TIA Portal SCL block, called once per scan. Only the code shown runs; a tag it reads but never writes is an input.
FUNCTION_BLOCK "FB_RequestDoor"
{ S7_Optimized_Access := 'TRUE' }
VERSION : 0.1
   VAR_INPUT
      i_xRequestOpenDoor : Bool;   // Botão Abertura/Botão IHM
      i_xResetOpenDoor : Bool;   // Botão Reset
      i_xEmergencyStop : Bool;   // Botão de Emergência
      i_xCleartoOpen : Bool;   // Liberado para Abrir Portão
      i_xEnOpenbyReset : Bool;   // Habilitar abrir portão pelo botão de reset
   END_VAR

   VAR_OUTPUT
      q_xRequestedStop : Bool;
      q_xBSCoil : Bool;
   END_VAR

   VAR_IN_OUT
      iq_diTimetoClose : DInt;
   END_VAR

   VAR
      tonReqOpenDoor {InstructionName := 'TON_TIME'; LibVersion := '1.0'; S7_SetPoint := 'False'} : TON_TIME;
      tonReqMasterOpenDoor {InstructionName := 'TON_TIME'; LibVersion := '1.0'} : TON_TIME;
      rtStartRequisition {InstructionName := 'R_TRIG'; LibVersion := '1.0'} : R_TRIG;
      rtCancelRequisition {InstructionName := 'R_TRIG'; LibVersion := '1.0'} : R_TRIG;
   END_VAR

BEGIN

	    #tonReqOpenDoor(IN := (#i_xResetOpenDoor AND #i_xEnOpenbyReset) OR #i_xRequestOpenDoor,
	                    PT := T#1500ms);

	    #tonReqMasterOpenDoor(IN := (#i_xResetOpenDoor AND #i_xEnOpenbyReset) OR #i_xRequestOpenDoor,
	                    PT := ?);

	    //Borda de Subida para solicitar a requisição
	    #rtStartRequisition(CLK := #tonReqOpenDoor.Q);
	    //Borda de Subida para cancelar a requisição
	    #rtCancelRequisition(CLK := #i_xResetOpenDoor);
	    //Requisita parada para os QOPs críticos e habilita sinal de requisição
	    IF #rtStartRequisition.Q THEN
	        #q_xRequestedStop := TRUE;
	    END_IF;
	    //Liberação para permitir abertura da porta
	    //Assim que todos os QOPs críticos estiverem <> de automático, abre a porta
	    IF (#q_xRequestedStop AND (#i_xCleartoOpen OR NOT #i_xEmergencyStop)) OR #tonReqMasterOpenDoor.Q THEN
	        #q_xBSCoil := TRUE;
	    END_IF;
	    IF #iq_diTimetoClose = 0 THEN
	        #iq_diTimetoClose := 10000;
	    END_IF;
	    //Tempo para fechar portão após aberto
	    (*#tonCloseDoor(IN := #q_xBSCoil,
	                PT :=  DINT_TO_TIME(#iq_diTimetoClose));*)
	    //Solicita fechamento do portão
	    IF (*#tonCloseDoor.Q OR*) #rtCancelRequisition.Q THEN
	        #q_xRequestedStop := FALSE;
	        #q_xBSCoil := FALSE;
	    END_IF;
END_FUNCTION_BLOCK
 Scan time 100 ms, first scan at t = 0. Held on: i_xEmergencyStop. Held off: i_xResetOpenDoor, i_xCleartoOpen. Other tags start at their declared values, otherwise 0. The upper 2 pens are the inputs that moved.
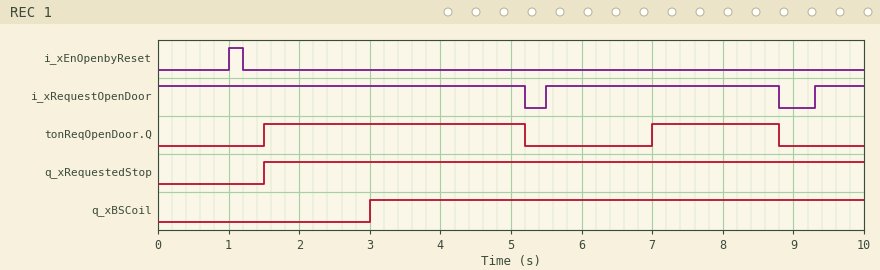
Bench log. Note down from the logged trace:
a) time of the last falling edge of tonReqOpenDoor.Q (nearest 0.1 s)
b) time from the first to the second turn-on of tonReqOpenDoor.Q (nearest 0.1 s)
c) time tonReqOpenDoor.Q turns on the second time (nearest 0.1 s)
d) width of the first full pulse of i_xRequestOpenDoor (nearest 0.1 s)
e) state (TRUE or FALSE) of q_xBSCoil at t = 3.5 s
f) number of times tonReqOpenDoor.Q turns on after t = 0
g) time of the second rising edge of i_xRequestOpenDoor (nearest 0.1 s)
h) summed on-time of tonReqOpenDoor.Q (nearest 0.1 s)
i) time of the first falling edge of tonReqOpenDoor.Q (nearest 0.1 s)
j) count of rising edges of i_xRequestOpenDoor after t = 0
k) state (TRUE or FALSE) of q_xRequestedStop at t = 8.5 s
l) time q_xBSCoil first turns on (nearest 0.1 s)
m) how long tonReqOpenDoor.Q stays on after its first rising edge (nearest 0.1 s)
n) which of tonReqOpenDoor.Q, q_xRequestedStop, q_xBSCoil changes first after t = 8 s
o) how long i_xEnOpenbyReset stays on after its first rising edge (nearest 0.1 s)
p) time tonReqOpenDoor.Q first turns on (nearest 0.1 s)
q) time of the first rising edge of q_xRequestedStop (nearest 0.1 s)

8.8 s
5.5 s
7.0 s
3.3 s
TRUE
2
9.3 s
5.5 s
5.2 s
2
TRUE
3.0 s
3.7 s
tonReqOpenDoor.Q
0.2 s
1.5 s
1.5 s
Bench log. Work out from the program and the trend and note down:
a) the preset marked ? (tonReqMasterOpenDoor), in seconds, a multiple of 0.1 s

3.0 s
